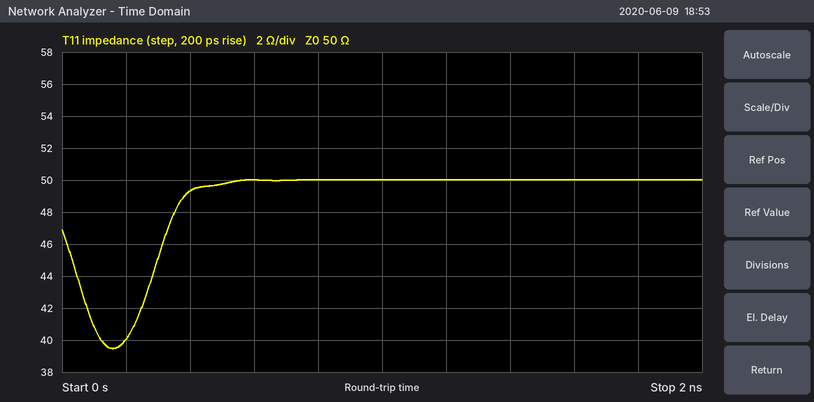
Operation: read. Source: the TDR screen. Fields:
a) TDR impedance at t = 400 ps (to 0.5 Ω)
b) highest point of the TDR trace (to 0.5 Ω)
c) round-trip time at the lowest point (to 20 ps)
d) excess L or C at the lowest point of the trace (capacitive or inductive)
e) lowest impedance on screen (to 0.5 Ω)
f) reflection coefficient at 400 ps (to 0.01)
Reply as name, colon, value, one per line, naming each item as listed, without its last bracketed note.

TDR impedance at t = 400 ps: 49.5 Ω
highest point of the TDR trace: 50.0 Ω
round-trip time at the lowest point: 160 ps
excess L or C at the lowest point of the trace: capacitive
lowest impedance on screen: 39.5 Ω
reflection coefficient at 400 ps: -0.01
